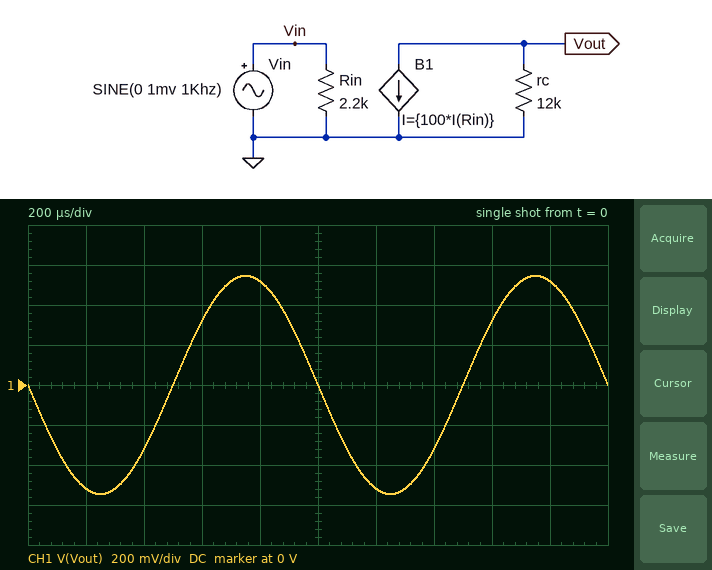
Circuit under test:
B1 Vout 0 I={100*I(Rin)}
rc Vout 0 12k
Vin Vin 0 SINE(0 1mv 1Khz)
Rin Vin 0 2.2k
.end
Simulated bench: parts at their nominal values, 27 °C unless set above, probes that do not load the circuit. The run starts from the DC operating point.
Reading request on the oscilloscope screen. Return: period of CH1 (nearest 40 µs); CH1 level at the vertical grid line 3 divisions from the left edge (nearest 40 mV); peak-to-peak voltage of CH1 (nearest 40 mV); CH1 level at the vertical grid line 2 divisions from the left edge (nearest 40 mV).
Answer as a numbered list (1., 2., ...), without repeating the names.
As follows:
1. 1.00 ms
2. 320 mV
3. 1.08 V
4. -320 mV
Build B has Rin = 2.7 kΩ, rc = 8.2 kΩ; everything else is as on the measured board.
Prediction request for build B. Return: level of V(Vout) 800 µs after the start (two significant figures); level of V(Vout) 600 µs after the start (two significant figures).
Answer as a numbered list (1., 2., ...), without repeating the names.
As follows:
1. 290 mV
2. 180 mV
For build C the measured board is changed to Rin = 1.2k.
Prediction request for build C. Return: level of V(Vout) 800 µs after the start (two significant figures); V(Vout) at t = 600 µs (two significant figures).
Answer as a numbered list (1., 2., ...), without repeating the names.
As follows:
1. 950 mV
2. 590 mV
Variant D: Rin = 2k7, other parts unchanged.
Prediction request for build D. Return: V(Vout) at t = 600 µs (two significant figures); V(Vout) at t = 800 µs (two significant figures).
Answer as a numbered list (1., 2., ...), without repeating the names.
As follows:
1. 260 mV
2. 420 mV
